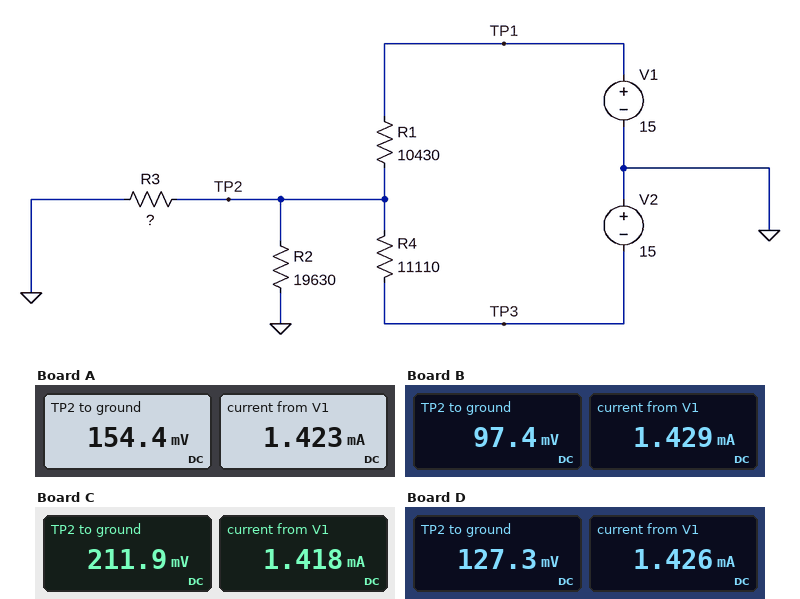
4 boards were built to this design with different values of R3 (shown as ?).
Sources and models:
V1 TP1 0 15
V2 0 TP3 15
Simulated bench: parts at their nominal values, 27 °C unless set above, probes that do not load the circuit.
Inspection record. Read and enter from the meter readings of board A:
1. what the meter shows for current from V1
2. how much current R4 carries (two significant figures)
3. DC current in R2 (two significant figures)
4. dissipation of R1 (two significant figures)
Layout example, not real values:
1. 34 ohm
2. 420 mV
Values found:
1. 1.423 mA
2. 1.4 mA
3. 7.9 µA
4. 21 mW
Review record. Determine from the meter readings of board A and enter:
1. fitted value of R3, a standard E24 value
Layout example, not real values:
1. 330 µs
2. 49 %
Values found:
1. 3 kΩ
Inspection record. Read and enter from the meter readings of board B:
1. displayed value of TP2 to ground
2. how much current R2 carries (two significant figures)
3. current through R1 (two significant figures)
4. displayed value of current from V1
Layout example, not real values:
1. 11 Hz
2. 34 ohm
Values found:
1. 97.4 mV
2. 5.0 µA
3. 1.4 mA
4. 1.429 mA
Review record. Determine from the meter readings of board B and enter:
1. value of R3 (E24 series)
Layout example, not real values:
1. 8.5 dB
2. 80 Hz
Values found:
1. 1.5 kΩ
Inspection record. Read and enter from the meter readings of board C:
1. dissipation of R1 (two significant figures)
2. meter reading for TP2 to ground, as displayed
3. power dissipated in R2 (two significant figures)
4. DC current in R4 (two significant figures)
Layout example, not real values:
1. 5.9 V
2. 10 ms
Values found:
1. 21 mW
2. 211.9 mV
3. 2.3 µW
4. 1.4 mA
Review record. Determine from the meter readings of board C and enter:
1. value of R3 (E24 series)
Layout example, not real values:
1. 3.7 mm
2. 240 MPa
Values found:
1. 5.6 kΩ
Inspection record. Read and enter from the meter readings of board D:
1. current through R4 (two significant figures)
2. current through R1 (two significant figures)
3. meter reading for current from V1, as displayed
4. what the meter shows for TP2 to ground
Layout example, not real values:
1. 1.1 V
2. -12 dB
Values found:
1. 1.4 mA
2. 1.4 mA
3. 1.426 mA
4. 127.3 mV
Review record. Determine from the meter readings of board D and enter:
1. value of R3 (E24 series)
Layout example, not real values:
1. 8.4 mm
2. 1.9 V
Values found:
1. 2.2 kΩ
